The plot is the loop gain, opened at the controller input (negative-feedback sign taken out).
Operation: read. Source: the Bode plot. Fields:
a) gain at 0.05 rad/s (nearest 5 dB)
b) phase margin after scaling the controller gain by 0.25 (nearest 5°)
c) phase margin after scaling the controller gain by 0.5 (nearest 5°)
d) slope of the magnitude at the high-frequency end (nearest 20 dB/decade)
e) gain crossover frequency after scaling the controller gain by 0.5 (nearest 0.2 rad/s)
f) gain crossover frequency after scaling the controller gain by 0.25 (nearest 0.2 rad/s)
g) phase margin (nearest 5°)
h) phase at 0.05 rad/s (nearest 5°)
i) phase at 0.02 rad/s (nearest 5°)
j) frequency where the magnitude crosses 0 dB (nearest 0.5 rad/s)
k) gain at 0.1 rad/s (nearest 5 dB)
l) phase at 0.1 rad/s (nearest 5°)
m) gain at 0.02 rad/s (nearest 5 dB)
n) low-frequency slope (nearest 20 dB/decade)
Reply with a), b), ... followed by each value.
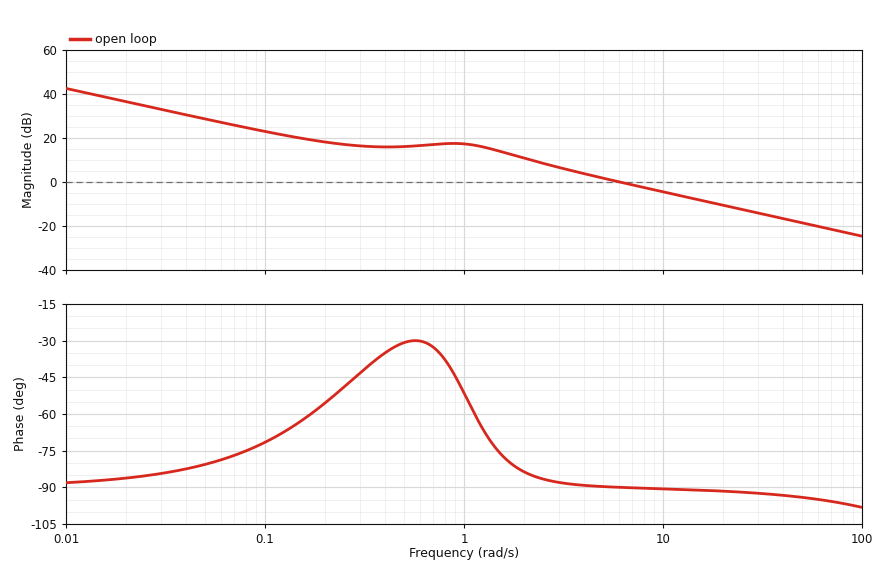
a) 30 dB
b) 100°
c) 90°
d) -20 dB/decade
e) 3.2 rad/s
f) 1.8 rad/s
g) 90°
h) -80°
i) -85°
j) 6.0 rad/s
k) 25 dB
l) -70°
m) 35 dB
n) -20 dB/decade
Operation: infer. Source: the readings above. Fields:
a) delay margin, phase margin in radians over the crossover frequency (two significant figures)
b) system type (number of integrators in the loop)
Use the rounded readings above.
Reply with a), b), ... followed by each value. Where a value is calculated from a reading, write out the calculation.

a) 90 × π / 180 / 6 = 0.26 s
b) 1
